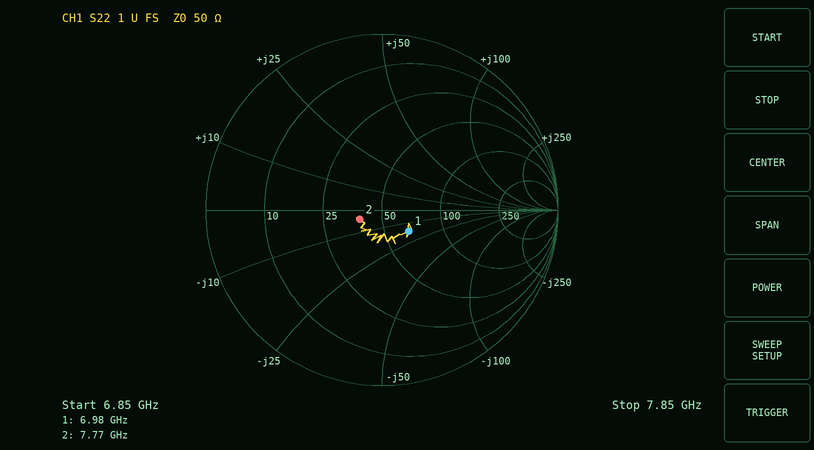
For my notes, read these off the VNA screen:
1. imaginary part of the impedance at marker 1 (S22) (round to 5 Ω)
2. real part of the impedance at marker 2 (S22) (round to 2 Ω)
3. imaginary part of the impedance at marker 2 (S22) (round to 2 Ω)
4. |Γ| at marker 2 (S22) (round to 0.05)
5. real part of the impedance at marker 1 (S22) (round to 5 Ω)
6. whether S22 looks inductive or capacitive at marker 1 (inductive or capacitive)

-15 Ω
38 Ω
-4 Ω
0.15
65 Ω
capacitive
